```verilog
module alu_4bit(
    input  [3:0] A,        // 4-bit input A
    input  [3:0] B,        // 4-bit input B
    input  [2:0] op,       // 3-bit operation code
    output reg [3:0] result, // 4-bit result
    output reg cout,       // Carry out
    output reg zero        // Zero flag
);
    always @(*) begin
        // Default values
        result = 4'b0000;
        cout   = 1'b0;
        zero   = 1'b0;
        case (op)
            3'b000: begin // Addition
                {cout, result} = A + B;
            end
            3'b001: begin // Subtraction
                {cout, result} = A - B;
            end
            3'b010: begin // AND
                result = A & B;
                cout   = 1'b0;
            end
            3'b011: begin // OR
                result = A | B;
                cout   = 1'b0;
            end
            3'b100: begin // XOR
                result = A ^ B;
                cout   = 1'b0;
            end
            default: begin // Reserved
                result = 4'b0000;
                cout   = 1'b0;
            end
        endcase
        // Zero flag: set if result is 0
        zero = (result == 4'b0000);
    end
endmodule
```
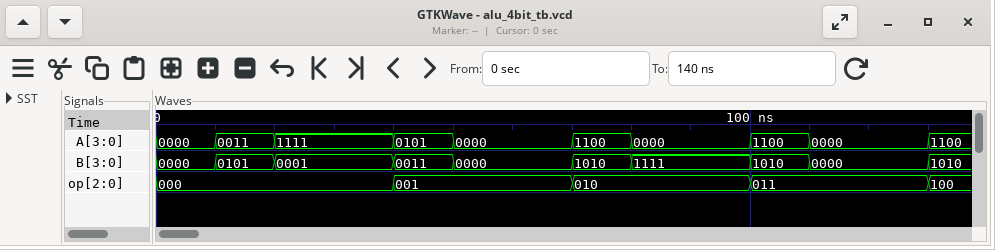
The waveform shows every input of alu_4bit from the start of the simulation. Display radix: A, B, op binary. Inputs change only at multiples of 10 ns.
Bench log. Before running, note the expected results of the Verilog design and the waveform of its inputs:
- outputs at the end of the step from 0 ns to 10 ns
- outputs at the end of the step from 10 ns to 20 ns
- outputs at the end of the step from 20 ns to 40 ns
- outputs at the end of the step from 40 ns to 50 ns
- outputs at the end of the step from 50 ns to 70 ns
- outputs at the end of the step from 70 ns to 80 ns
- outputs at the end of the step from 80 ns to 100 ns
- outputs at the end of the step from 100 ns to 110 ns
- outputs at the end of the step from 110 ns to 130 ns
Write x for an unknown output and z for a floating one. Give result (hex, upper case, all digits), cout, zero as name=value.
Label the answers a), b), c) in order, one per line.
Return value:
a) result=0, cout=0, zero=1
b) result=8, cout=0, zero=0
c) result=0, cout=1, zero=1
d) result=2, cout=0, zero=0
e) result=0, cout=0, zero=1
f) result=8, cout=0, zero=0
g) result=0, cout=0, zero=1
h) result=E, cout=0, zero=0
i) result=0, cout=0, zero=1
